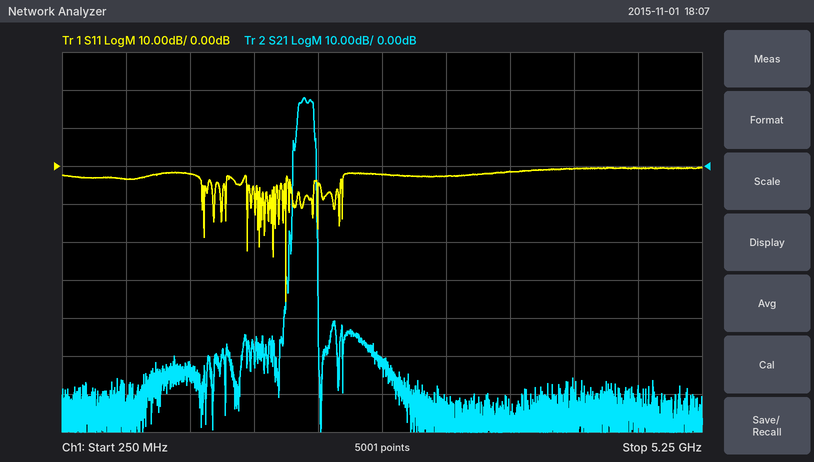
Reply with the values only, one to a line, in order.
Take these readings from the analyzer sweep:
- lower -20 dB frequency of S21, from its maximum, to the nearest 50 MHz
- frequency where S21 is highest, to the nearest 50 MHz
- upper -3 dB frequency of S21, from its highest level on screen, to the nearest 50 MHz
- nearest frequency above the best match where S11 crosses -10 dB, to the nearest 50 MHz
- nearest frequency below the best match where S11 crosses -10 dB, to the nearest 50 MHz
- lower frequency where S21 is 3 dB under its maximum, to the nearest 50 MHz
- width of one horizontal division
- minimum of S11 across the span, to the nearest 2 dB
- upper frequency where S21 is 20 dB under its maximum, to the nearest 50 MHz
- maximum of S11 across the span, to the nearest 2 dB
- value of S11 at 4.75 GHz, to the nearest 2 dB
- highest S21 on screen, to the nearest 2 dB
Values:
2.05 GHz
2.15 GHz
2.20 GHz
2.00 GHz
2.00 GHz
2.10 GHz
500 MHz
-36 dB
2.25 GHz
0 dB
0 dB
18 dB
